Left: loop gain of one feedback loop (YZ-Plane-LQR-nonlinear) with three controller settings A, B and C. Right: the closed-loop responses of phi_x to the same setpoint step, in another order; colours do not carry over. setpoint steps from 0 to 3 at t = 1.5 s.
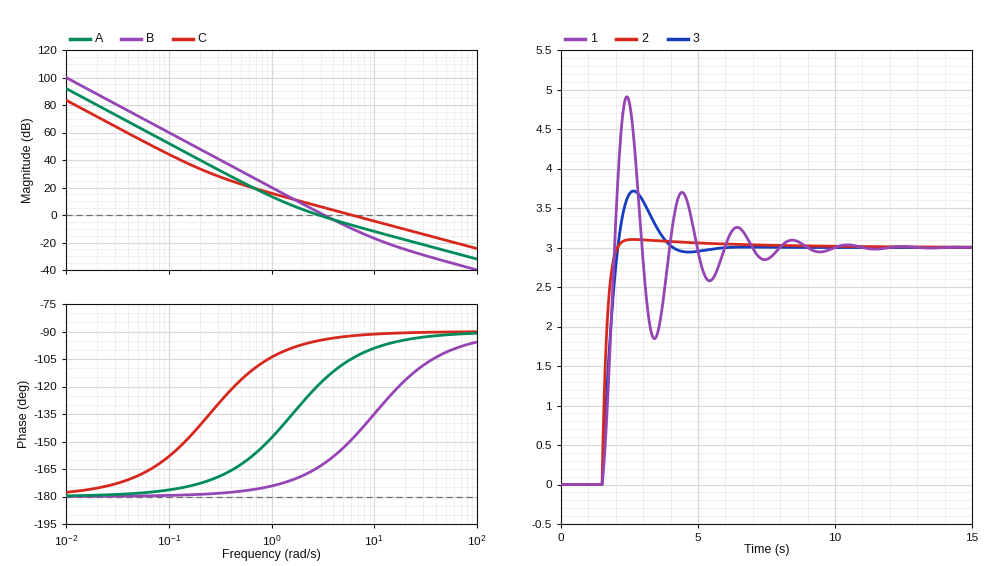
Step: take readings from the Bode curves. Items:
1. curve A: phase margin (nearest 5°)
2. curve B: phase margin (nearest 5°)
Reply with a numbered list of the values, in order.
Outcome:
1. 60°
2. 20°
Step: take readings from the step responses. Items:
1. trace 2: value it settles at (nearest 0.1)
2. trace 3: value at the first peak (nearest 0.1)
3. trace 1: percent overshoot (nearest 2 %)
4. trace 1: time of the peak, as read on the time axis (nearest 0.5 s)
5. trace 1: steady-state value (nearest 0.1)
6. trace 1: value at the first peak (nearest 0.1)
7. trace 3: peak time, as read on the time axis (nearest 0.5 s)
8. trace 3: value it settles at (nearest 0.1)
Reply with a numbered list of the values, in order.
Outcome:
1. 3.0
2. 3.7
3. 64 %
4. 2.5 s
5. 3.0
6. 4.9
7. 2.5 s
8. 3.0
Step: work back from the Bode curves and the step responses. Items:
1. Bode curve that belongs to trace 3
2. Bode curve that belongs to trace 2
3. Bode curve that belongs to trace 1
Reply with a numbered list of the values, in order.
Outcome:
1. A
2. C
3. B
